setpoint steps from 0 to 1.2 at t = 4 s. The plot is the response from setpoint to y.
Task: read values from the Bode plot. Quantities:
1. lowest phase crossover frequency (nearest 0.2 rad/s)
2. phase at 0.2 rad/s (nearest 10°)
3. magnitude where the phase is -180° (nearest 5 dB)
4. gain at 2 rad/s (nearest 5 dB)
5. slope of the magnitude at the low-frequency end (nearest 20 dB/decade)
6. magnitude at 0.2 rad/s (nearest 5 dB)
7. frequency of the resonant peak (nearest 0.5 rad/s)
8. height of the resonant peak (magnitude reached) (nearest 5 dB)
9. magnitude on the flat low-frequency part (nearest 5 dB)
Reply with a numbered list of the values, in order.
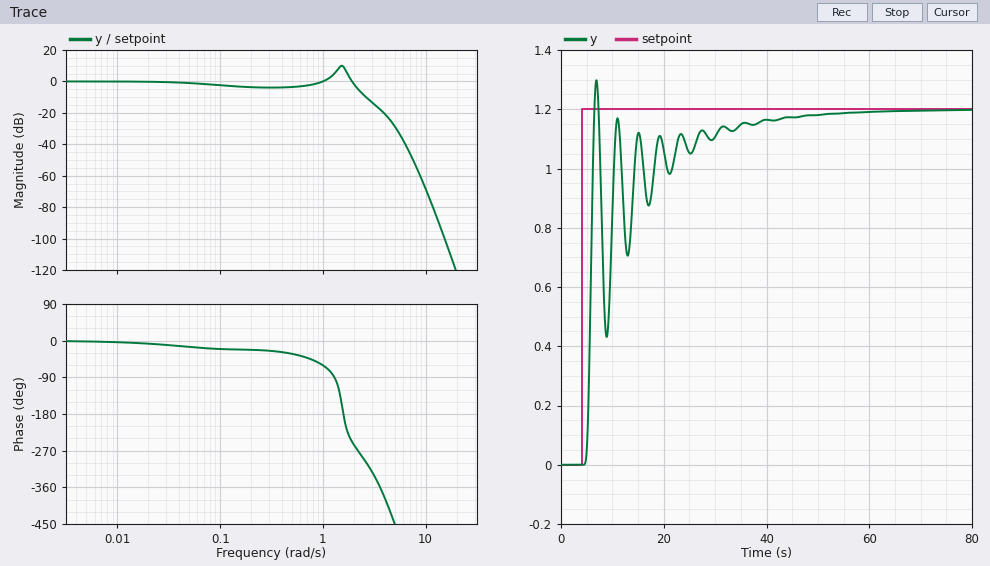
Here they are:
1. 1.6 rad/s
2. -20°
3. 10 dB
4. 0 dB
5. 0 dB/decade
6. -5 dB
7. 1.5 rad/s
8. 10 dB
9. 0 dB
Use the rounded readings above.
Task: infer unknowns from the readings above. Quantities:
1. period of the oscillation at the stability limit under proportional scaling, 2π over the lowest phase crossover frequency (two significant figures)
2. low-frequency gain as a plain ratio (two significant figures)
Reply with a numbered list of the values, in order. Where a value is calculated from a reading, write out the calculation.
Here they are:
1. 2π / 1.6 = 3.9 s
2. 10^(0 / 20) = 1.0
